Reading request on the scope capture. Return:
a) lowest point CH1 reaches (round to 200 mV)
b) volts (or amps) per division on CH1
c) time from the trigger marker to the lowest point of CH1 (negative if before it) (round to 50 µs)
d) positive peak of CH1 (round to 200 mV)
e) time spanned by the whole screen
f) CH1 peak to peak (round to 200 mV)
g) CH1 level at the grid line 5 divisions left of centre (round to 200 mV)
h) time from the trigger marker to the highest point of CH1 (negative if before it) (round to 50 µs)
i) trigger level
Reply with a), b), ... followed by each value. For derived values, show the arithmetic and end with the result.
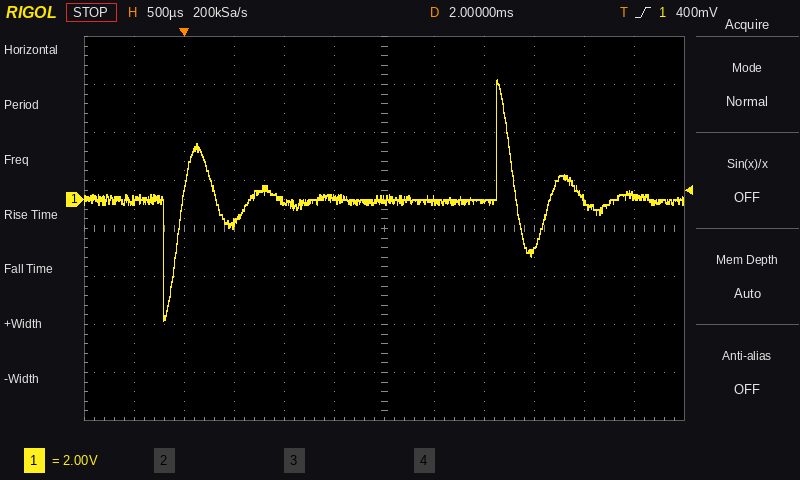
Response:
a) -5.0 V
b) 2 V
c) -200 µs
d) 5.0 V
e) 6 ms
f) 5.0 V − (-5.0 V) = 10.0 V
g) 0.0 V
h) +3.15 ms
i) 400 mV
